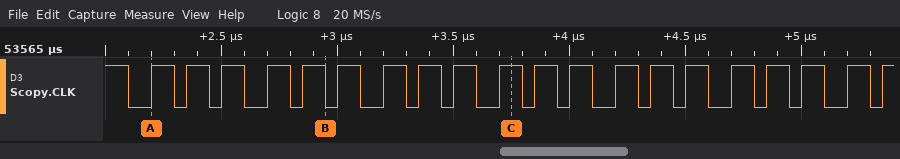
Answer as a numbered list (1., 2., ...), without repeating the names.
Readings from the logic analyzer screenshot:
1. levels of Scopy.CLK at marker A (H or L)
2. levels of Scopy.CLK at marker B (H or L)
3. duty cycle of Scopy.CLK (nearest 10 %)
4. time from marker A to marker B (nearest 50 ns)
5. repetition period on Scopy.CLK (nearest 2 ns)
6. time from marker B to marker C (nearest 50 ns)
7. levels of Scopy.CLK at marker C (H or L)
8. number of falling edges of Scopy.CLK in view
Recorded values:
1. Scopy.CLK=H
2. Scopy.CLK=L
3. 60 %
4. 750 ns
5. 166 ns
6. 800 ns
7. Scopy.CLK=H
8. 20
